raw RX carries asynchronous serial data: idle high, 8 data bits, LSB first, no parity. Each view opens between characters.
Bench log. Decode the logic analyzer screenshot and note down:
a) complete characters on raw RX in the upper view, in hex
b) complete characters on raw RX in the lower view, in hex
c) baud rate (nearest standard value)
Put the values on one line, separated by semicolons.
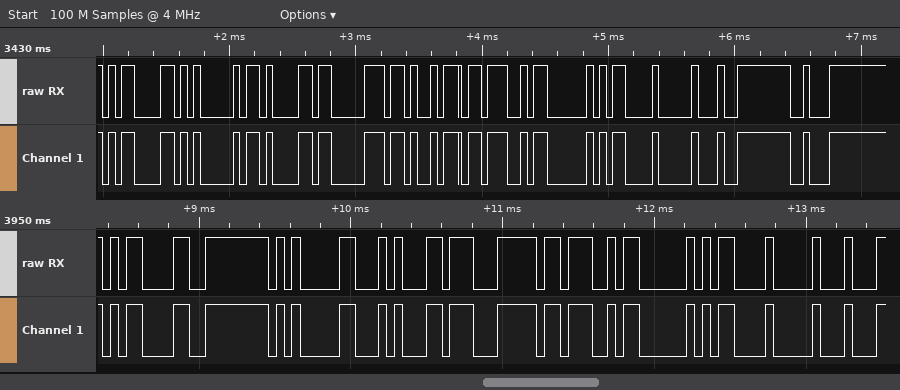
0D, 05, 0B, 83, 4B, 3B, 03, 0D, 10, FE, E2; 0D, FE, 05, 14, C7, 3B, 03, 0D, 10; 19200 baud
